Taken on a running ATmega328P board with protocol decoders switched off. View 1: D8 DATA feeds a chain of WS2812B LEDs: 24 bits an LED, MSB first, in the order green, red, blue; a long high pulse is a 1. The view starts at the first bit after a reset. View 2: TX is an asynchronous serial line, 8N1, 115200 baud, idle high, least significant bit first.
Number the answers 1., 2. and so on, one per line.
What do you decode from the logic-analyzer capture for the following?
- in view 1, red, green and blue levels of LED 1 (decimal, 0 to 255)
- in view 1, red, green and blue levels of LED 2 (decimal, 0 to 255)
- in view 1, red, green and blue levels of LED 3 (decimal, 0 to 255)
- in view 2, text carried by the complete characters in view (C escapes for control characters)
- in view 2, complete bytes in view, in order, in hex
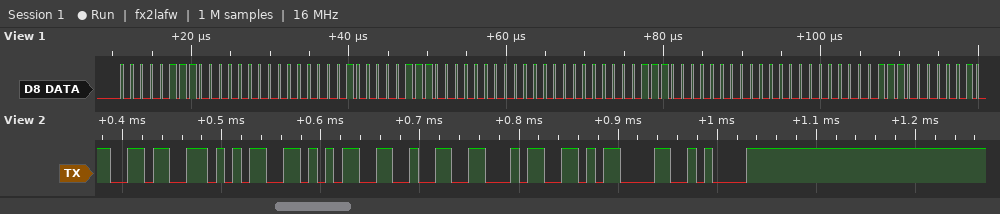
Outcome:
1. 0, 7, 1
2. 0, 7, 0
3. 0, 7, 0
4. "65524\r\n"
5. 36 35 35 32 34 0D 0A
